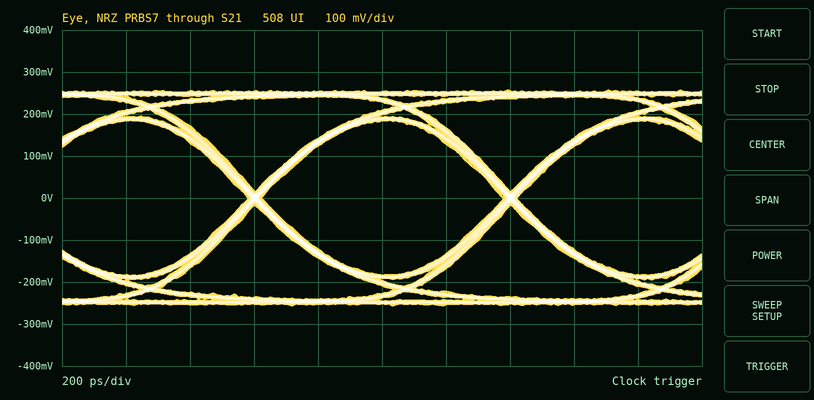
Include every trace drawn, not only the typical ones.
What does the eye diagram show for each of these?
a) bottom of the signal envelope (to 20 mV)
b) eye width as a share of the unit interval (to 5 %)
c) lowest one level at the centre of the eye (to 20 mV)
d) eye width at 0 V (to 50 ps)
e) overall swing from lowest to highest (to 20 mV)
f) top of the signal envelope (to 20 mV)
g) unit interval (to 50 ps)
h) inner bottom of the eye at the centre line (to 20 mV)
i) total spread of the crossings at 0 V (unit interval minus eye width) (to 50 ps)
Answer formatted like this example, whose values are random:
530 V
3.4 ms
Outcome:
-260 mV
95 %
180 mV
750 ps
520 mV
260 mV
800 ps
-180 mV
50 ps
